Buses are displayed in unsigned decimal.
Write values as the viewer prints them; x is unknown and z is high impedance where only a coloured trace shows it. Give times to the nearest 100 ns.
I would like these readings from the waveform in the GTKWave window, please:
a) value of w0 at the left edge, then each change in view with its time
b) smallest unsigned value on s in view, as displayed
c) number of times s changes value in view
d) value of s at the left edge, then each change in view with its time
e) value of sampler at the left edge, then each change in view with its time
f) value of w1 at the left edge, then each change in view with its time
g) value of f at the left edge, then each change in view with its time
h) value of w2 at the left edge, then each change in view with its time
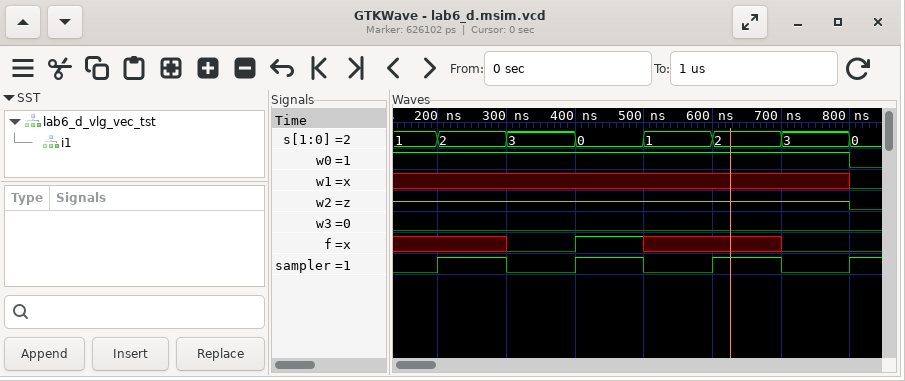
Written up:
1, 0 at 800 ns
0
7
1, 2 at 200 ns, 3 at 300 ns, 0 at 400 ns, 1 at 500 ns, 2 at 600 ns, 3 at 700 ns, 0 at 800 ns
0, 1 at 200 ns, 0 at 300 ns, 1 at 400 ns, 0 at 500 ns, 1 at 600 ns, 0 at 700 ns, 1 at 800 ns
x, 0 at 800 ns
x, 0 at 300 ns, 1 at 400 ns, x at 500 ns, 0 at 700 ns
z, 0 at 800 ns
